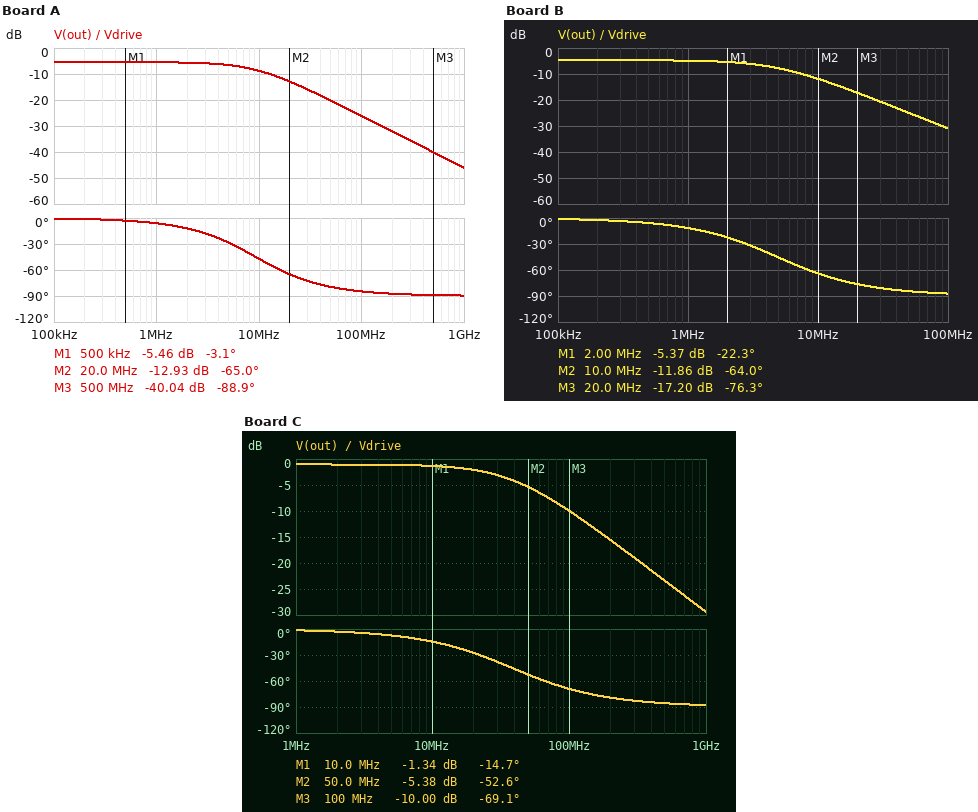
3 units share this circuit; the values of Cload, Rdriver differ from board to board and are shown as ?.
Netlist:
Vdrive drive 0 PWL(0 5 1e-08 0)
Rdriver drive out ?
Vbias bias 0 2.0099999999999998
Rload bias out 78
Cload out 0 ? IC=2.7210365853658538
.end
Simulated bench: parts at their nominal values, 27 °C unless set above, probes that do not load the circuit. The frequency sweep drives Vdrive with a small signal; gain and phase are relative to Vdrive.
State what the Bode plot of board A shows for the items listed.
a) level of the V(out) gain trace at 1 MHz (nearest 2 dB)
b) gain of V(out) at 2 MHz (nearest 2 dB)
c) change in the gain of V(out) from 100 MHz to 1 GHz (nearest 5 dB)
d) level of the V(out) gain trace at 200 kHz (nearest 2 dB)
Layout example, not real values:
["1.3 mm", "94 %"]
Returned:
["-6 dB", "-6 dB", "-20 dB", "-6 dB"]
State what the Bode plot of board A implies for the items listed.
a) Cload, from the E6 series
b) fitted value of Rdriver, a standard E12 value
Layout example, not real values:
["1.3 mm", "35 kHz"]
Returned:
["470 pF", "68 Ω"]
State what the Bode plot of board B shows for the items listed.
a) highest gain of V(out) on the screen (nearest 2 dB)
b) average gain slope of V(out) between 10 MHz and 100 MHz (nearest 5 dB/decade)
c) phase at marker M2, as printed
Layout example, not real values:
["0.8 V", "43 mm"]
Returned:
["-4 dB", "-20 dB/decade", "-64.0 deg"]
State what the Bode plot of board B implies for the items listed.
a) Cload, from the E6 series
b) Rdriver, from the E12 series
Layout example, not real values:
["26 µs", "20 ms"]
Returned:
["1 nF", "56 Ω"]
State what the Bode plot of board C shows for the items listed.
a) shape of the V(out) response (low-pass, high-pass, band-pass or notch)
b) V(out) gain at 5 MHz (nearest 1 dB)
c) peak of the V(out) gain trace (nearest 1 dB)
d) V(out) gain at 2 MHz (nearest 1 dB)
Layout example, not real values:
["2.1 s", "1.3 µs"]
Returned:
["low-pass", "-1 dB", "-1 dB", "-1 dB"]
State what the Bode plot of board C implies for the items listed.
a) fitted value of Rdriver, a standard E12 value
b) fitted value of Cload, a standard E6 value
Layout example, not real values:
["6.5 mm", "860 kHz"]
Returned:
["10 Ω", "470 pF"]
